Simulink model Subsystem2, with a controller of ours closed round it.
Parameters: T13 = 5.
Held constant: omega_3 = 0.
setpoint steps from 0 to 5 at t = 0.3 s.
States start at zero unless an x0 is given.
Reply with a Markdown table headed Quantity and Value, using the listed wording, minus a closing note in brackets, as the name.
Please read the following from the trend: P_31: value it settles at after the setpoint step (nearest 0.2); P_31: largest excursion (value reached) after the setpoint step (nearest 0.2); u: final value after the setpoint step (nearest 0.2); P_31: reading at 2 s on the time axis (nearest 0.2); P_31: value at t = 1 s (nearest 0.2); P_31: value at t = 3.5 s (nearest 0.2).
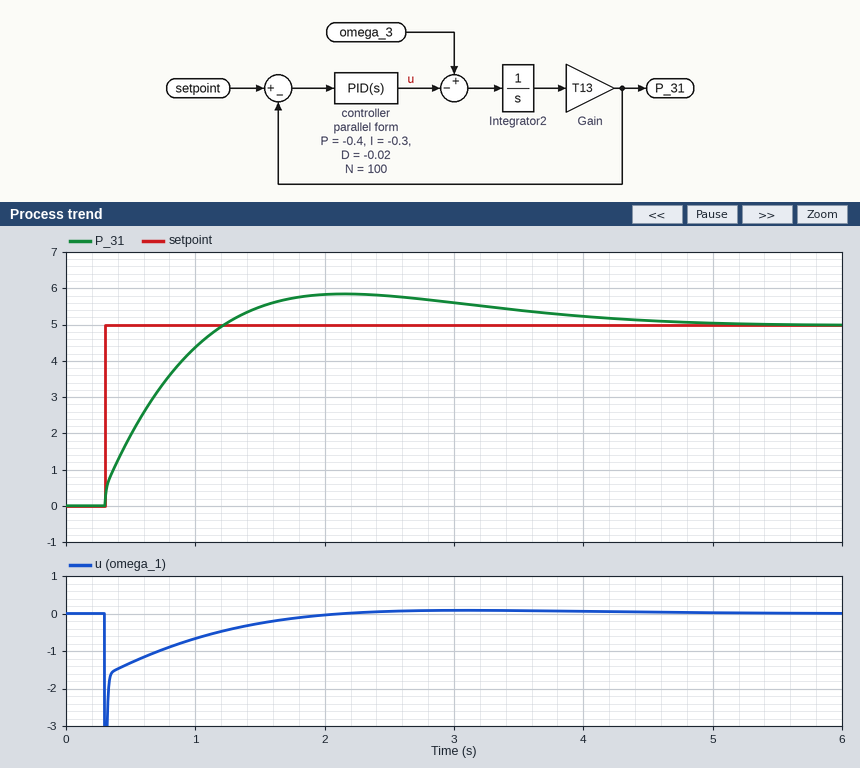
| Quantity | Value |
|---|---|
| P_31: value it settles at after the setpoint step | 5.0 |
| P_31: largest excursion (value reached) after the setpoint step | 5.8 |
| u: final value after the setpoint step | 0.0 |
| P_31: reading at 2 s on the time axis | 5.8 |
| P_31: value at t = 1 s | 4.4 |
| P_31: value at t = 3.5 s | 5.4 |
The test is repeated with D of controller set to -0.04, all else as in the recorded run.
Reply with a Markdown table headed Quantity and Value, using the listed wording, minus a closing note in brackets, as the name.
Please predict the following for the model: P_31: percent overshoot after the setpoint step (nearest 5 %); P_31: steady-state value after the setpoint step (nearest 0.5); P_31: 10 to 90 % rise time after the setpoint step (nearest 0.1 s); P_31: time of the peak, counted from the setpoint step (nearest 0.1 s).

| Quantity | Value |
|---|---|
| P_31: percent overshoot after the setpoint step | 15 % |
| P_31: steady-state value after the setpoint step | 5.0 |
| P_31: 10 to 90 % rise time after the setpoint step | 0.8 s |
| P_31: time of the peak, counted from the setpoint step | 2.0 s |
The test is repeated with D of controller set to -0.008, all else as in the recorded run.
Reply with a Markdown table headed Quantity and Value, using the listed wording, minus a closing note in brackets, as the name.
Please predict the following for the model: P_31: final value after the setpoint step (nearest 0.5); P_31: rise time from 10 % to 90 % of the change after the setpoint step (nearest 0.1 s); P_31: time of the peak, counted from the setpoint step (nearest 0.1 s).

| Quantity | Value |
|---|---|
| P_31: final value after the setpoint step | 5.0 |
| P_31: rise time from 10 % to 90 % of the change after the setpoint step | 0.7 s |
| P_31: time of the peak, counted from the setpoint step | 1.8 s |
